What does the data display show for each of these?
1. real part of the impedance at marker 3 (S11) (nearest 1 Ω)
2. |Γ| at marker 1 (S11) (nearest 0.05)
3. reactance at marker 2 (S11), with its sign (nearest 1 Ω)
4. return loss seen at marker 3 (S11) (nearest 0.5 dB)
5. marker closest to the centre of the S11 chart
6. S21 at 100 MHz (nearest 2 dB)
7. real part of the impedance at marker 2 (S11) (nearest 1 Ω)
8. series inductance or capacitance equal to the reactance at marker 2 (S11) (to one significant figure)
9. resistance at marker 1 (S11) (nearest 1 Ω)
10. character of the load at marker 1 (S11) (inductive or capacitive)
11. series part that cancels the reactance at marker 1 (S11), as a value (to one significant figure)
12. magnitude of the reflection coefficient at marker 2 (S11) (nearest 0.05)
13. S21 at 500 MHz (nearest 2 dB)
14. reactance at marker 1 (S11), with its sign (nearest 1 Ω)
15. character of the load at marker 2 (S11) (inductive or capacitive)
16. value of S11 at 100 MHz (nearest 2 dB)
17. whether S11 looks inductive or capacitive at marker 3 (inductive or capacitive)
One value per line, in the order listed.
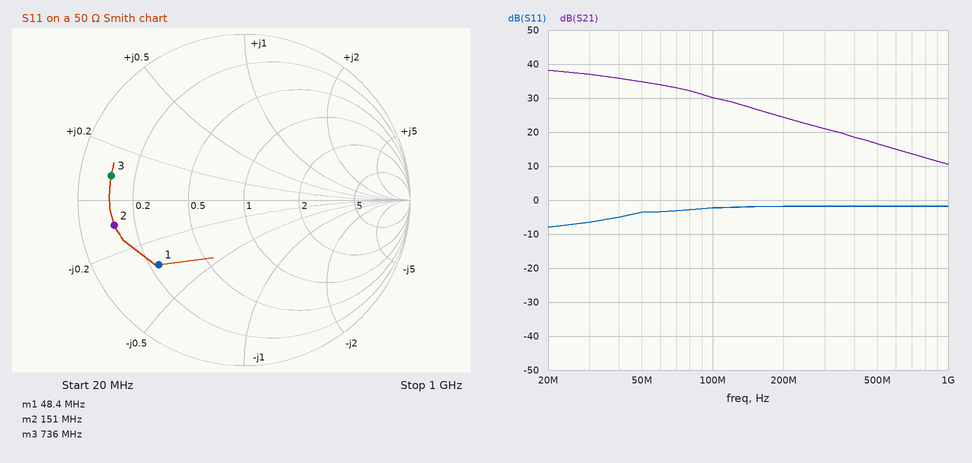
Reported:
5 Ω
0.65
-5 Ω
2.0 dB
marker 1
30 dB
6 Ω
200 pF
12 Ω
capacitive
50 nH
0.80
16 dB
-16 Ω
capacitive
-2 dB
inductive
